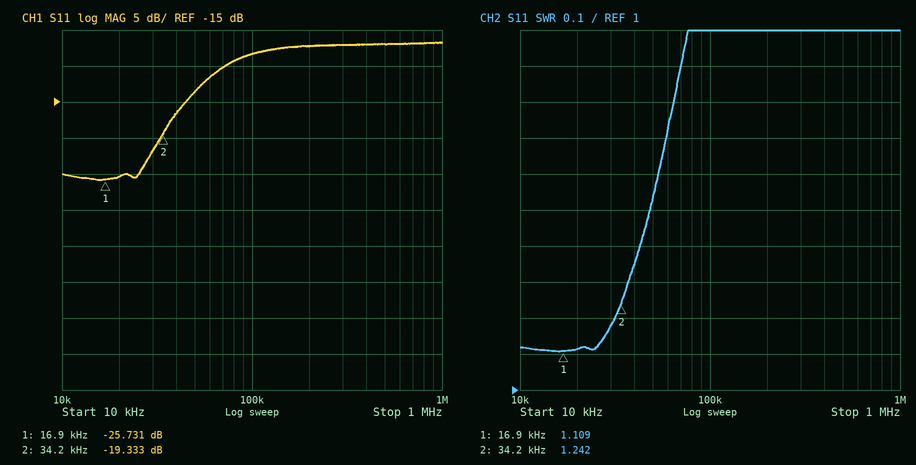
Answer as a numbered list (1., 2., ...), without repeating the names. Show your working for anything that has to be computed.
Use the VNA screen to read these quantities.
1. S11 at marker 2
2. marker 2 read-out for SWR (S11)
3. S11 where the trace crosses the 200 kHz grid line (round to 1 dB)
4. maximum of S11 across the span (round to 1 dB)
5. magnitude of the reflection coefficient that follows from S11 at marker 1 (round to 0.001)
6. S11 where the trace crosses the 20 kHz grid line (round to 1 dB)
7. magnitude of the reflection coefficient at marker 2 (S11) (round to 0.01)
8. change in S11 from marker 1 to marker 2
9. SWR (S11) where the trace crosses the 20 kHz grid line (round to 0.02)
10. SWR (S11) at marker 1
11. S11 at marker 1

1. -19.333 dB
2. 1.242
3. -7 dB
4. -7 dB
5. 10^(-25.731/20) ≈ 0.052
6. -25 dB
7. 10^(-19.333/20) ≈ 0.11
8. -19.333 − (-25.731) = 6.398 dB
9. 1.12
10. 1.109
11. -25.731 dB
